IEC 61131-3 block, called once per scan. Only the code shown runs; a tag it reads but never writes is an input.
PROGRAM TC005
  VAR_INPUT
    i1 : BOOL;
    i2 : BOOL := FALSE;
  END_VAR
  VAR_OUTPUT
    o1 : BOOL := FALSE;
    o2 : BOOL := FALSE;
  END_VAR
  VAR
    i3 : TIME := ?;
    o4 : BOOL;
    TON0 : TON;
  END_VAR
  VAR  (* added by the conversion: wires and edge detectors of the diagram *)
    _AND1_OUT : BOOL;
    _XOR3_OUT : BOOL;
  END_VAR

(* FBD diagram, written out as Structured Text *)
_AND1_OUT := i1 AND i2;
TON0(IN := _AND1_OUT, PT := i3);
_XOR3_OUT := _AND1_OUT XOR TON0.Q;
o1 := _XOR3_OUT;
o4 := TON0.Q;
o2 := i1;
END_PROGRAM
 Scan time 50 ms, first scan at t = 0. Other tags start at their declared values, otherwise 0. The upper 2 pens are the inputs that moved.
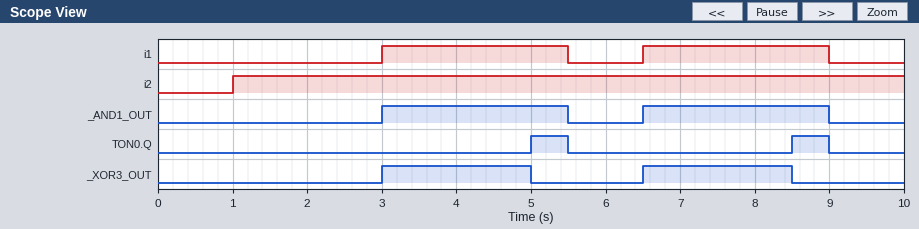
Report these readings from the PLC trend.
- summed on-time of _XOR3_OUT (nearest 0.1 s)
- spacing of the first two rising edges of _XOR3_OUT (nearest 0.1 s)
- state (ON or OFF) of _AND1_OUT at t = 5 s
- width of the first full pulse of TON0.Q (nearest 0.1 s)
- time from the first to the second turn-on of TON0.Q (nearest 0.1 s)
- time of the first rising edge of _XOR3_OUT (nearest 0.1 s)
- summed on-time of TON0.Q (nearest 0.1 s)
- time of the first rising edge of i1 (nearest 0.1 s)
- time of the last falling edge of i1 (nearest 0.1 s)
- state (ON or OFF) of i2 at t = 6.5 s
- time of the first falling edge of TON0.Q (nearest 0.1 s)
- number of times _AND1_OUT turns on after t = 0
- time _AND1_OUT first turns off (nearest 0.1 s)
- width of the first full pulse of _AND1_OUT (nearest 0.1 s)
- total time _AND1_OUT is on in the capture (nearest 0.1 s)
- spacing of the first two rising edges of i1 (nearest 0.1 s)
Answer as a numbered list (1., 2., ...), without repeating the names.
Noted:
1. 4.0 s
2. 3.5 s
3. ON
4. 0.5 s
5. 3.5 s
6. 3.0 s
7. 1.0 s
8. 3.0 s
9. 9.0 s
10. ON
11. 5.5 s
12. 2
13. 5.5 s
14. 2.5 s
15. 5.0 s
16. 3.5 s
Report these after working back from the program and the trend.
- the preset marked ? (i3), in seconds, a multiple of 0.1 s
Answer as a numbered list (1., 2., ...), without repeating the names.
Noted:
1. 2.0 s
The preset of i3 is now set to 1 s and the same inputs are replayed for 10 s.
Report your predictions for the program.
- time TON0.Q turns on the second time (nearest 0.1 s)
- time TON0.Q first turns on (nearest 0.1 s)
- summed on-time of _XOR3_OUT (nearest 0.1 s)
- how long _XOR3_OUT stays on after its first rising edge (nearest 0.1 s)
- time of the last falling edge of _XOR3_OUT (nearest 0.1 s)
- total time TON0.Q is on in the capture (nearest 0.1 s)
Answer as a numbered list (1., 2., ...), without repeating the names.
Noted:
1. 7.5 s
2. 4.0 s
3. 2.0 s
4. 1.0 s
5. 7.5 s
6. 3.0 s
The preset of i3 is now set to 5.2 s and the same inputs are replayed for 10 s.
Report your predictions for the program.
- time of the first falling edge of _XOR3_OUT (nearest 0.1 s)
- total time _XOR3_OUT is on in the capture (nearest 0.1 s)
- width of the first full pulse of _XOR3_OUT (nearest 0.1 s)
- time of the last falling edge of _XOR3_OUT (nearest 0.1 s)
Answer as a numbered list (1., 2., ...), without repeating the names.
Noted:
1. 5.5 s
2. 5.0 s
3. 2.5 s
4. 9.0 s
